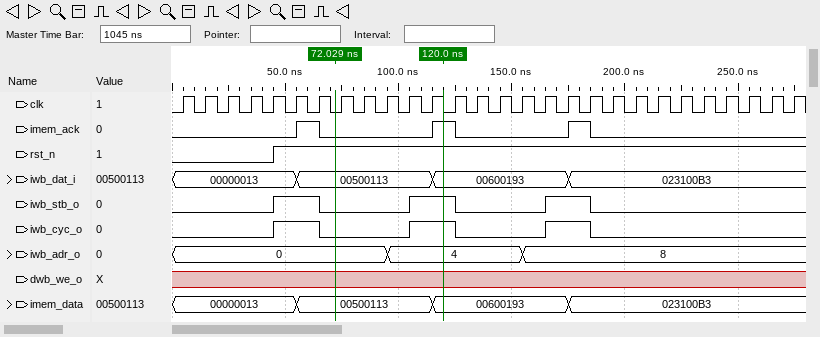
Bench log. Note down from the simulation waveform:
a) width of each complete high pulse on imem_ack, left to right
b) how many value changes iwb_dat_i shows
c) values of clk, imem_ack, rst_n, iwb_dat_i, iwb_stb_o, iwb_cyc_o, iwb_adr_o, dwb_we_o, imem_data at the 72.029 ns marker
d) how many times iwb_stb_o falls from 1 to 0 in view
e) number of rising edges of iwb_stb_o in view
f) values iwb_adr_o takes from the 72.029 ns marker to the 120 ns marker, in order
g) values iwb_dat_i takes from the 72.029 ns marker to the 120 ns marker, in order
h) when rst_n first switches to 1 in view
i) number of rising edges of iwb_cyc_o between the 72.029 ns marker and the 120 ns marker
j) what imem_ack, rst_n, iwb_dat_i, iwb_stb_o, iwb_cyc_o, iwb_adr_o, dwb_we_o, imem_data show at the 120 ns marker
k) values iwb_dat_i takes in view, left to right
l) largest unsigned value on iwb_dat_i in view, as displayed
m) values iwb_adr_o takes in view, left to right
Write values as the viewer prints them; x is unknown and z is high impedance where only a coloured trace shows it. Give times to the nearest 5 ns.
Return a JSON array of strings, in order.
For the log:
["10 ns, 10 ns, 10 ns", "3", "clk=0, imem_ack=0, rst_n=1, iwb_dat_i=00500113, iwb_stb_o=0, iwb_cyc_o=0, iwb_adr_o=0, dwb_we_o=x, imem_data=00500113", "3", "3", "0, 4", "00500113, 00600193", "45 ns", "1", "imem_ack=1, rst_n=1, iwb_dat_i=00600193, iwb_stb_o=1, iwb_cyc_o=1, iwb_adr_o=4, dwb_we_o=x, imem_data=00600193", "00000013, 00500113, 00600193, 023100B3", "023100B3", "0, 4, 8"]
